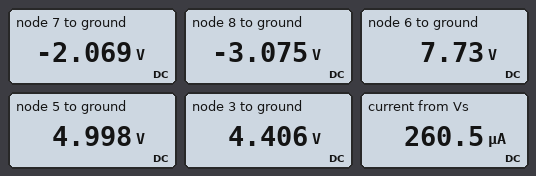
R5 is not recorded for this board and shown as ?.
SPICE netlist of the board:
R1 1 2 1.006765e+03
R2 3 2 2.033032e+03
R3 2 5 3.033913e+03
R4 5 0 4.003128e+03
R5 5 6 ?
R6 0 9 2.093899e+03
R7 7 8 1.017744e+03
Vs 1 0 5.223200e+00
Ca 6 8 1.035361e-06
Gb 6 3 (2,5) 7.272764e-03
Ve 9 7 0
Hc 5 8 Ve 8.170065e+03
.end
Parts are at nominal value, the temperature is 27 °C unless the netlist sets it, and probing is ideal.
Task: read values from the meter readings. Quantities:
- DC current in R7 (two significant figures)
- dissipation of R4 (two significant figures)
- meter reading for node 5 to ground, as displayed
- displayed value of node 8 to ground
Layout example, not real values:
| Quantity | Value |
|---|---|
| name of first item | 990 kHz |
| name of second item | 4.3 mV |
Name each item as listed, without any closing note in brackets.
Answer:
| Quantity | Value |
|---|---|
| DC current in R7 | 990 µA |
| dissipation of R4 | 6.2 mW |
| meter reading for node 5 to ground, as displayed | 4.998 V |
| displayed value of node 8 to ground | -3.075 V |
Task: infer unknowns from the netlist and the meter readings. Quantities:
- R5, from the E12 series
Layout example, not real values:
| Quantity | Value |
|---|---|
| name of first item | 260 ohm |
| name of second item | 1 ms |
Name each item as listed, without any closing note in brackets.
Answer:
| Quantity | Value |
|---|---|
| R5, from the E12 series | 10 kΩ |
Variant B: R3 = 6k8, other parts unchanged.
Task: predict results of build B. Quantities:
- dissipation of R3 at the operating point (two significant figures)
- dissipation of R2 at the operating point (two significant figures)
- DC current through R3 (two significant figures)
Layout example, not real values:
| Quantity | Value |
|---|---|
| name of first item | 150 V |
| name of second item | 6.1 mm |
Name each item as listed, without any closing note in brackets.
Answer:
| Quantity | Value |
|---|---|
| dissipation of R3 at the operating point | 200 nW |
| dissipation of R2 at the operating point | 140 µW |
| DC current through R3 | 5.4 µA |
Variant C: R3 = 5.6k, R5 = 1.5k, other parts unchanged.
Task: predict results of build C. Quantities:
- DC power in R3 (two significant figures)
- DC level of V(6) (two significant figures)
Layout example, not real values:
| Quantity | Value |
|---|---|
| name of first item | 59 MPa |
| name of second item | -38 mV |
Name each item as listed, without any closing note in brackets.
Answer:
| Quantity | Value |
|---|---|
| DC power in R3 | 240 nW |
| DC level of V(6) | 5.4 V |
